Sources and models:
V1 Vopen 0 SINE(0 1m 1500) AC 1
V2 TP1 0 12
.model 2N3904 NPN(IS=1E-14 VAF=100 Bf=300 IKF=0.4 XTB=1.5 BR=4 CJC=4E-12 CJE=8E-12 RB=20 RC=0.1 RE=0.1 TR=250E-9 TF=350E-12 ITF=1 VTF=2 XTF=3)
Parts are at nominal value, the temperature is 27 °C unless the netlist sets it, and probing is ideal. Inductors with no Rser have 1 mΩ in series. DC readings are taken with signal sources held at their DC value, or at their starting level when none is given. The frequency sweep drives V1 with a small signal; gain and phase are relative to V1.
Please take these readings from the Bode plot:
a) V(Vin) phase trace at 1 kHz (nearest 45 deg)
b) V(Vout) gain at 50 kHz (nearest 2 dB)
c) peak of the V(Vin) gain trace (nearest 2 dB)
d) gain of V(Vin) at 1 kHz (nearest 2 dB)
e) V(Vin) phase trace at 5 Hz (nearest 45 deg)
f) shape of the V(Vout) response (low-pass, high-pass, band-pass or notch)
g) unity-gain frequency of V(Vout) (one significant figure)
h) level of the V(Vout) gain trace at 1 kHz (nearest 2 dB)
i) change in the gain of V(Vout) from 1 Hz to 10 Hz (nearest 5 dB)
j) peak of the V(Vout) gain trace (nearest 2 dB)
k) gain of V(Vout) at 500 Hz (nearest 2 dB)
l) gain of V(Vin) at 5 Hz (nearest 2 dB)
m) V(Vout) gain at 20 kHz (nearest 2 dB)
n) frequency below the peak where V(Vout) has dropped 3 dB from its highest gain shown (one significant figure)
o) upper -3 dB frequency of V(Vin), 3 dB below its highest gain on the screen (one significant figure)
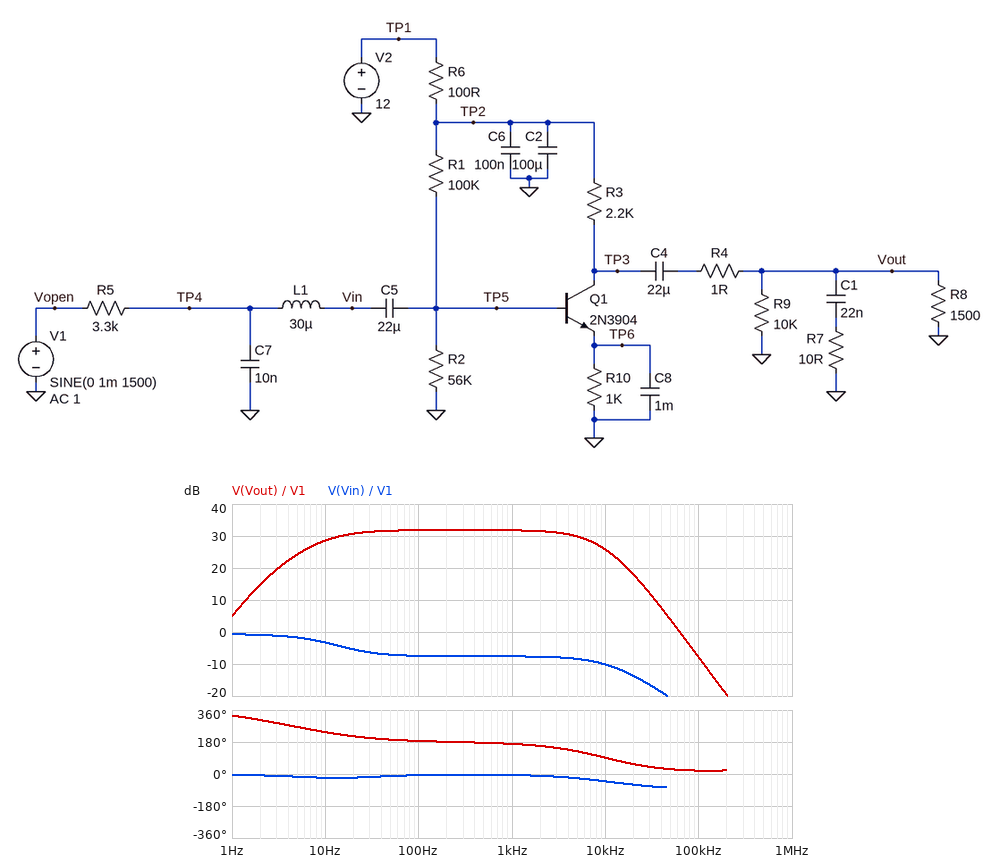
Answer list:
0 deg
4 dB
0 dB
-8 dB
0 deg
band-pass
60 kHz
32 dB
25 dB
32 dB
32 dB
-2 dB
18 dB
10 Hz
10 Hz
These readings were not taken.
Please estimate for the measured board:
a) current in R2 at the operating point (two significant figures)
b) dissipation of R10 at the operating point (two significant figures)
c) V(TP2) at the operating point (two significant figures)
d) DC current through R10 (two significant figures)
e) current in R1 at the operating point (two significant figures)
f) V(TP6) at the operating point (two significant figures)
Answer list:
68 µA
9.8 mW
12 V
3.1 mA
79 µA
3.1 V
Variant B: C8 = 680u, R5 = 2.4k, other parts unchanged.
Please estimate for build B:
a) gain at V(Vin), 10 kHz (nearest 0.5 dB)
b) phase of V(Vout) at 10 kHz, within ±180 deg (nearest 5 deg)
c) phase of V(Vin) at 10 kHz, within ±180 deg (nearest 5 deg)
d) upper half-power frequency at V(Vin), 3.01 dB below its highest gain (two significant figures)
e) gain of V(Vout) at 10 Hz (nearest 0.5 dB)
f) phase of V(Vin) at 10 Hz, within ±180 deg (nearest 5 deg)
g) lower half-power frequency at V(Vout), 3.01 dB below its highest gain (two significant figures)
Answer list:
-8.0 dB
95 deg
-35 deg
18 Hz
27.5 dB
-15 deg
17 Hz
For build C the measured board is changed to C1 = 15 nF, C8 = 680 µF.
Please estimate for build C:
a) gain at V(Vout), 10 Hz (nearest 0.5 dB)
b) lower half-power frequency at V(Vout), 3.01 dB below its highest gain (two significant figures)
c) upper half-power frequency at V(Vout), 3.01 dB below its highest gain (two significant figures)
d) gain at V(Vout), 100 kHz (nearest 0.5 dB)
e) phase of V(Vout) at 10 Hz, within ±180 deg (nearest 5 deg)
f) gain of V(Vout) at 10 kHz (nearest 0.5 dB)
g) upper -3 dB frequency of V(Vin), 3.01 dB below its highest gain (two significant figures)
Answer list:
27.0 dB
15 Hz
7.7 kHz
-4.5 dB
-115 deg
27.5 dB
13 Hz
